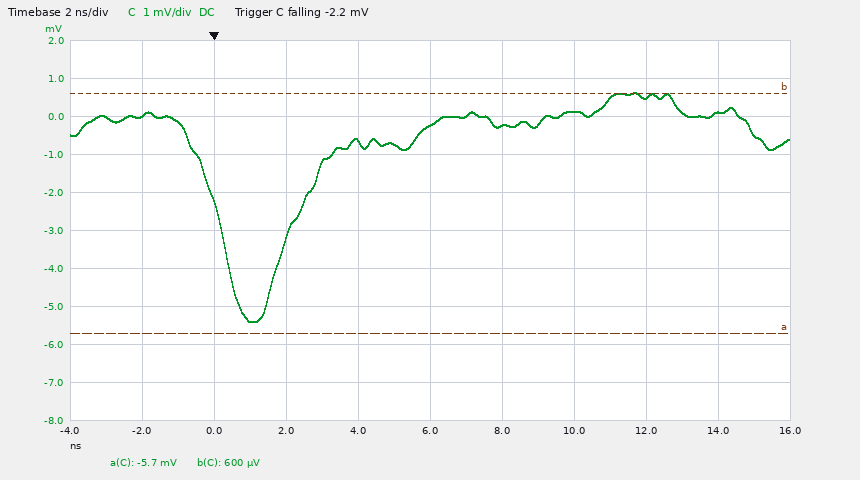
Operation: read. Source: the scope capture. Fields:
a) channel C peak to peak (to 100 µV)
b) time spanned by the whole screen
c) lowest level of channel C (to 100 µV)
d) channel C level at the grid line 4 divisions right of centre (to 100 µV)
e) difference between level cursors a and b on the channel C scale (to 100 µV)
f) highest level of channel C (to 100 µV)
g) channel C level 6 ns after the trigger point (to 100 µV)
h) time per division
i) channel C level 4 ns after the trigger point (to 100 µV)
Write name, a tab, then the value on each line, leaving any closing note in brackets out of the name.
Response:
channel C peak to peak	6.0 mV
time spanned by the whole screen	20 ns
lowest level of channel C	-5.4 mV
channel C level at the grid line 4 divisions right of centre	100 µV
difference between level cursors a and b on the channel C scale	6.3 mV
highest level of channel C	600 µV
channel C level 6 ns after the trigger point	-200 µV
time per division	2 ns
channel C level 4 ns after the trigger point	-700 µV
